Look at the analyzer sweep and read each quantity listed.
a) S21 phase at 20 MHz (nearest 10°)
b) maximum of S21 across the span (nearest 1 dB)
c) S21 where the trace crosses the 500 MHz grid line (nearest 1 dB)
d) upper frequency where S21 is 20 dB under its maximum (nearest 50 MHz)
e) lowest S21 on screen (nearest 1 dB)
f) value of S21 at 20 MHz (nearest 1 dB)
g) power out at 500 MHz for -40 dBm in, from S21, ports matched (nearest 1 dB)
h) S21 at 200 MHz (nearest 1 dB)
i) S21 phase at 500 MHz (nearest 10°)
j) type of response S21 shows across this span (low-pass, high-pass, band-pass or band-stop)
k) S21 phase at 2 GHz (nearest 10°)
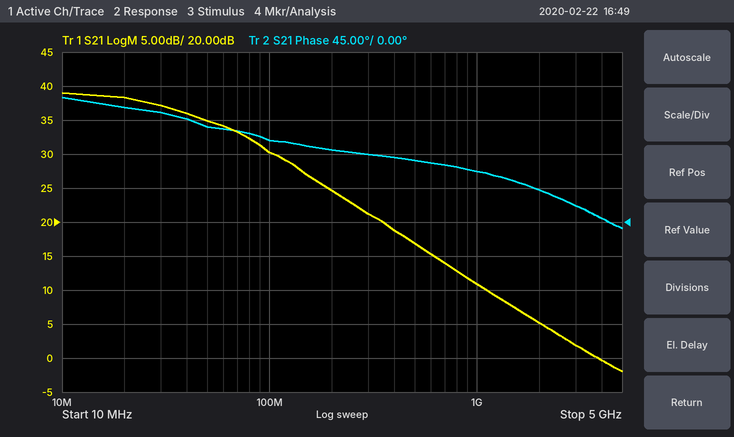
150°
39 dB
17 dB
400 MHz
-2 dB
38 dB
-23 dBm
25 dB
80°
low-pass
40°
